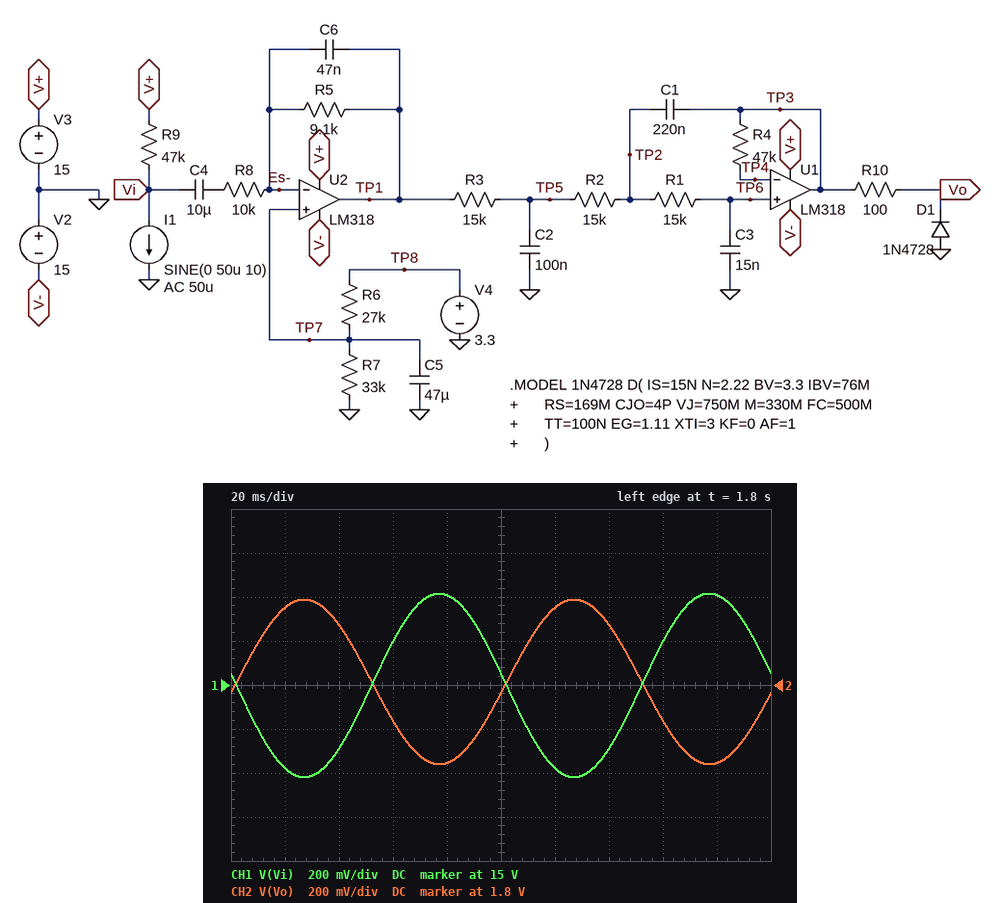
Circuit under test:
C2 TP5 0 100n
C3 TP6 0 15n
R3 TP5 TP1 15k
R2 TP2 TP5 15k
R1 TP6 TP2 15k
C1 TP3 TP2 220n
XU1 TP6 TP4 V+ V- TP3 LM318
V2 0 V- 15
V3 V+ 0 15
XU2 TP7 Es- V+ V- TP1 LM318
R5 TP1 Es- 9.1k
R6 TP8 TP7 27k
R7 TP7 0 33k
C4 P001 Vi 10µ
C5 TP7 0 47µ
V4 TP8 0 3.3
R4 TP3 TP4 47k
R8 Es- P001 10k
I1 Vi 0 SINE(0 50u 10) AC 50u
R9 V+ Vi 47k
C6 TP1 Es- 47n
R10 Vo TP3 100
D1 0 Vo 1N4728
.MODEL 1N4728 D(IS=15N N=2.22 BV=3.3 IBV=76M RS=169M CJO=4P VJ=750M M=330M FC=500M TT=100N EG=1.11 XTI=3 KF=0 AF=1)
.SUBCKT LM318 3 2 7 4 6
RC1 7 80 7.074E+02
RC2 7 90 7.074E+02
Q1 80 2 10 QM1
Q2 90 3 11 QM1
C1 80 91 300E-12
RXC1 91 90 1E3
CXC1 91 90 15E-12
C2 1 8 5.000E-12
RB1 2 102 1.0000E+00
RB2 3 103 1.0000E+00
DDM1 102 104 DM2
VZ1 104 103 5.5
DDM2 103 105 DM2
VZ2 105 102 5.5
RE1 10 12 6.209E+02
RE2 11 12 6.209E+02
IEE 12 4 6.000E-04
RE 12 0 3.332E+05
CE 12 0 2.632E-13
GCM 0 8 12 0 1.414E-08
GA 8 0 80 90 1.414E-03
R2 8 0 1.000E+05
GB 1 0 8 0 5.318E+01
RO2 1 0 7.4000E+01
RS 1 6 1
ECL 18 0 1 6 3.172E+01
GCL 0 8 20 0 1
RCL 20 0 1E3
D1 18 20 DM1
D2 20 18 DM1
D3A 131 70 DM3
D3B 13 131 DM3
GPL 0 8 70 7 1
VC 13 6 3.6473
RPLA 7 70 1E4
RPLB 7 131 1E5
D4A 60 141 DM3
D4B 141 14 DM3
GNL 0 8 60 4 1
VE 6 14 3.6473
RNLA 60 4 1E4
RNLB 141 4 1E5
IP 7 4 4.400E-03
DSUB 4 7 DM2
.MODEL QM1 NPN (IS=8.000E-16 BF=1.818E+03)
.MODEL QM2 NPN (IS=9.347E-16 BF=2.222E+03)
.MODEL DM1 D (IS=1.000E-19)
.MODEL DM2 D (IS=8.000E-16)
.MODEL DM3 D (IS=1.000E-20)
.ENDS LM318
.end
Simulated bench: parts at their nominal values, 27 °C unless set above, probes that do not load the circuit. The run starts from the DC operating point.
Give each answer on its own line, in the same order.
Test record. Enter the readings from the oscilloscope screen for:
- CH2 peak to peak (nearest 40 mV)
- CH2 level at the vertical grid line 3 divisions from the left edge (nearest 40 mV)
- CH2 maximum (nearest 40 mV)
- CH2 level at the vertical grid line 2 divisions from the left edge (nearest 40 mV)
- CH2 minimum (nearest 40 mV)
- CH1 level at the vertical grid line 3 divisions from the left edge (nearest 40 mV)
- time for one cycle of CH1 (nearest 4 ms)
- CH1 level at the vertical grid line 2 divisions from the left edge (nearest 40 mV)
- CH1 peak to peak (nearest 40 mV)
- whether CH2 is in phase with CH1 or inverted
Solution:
760 mV
1.64 V
2.20 V
2.08 V
1.44 V
15.20 V
100 ms
14.72 V
840 mV
inverted
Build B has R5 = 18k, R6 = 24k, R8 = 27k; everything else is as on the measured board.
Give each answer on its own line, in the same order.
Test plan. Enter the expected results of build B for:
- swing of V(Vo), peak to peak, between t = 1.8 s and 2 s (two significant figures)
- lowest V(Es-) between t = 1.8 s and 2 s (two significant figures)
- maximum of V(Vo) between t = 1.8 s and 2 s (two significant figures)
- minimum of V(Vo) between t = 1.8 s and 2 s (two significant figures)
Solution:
1.1 V
1.9 V
2.5 V
1.3 V
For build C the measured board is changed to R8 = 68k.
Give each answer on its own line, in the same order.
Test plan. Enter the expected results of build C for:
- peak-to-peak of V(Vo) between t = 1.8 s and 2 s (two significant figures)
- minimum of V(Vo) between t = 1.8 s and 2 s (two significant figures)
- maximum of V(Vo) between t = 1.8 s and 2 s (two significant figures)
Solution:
370 mV
1.6 V
2.0 V
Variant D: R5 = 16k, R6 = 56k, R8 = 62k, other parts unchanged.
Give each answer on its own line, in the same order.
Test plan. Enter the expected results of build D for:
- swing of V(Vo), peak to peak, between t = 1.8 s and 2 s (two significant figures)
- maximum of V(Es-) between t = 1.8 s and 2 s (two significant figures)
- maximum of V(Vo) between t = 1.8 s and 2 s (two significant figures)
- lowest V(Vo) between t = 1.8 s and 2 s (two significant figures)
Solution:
690 mV
1.2 V
1.6 V
880 mV
